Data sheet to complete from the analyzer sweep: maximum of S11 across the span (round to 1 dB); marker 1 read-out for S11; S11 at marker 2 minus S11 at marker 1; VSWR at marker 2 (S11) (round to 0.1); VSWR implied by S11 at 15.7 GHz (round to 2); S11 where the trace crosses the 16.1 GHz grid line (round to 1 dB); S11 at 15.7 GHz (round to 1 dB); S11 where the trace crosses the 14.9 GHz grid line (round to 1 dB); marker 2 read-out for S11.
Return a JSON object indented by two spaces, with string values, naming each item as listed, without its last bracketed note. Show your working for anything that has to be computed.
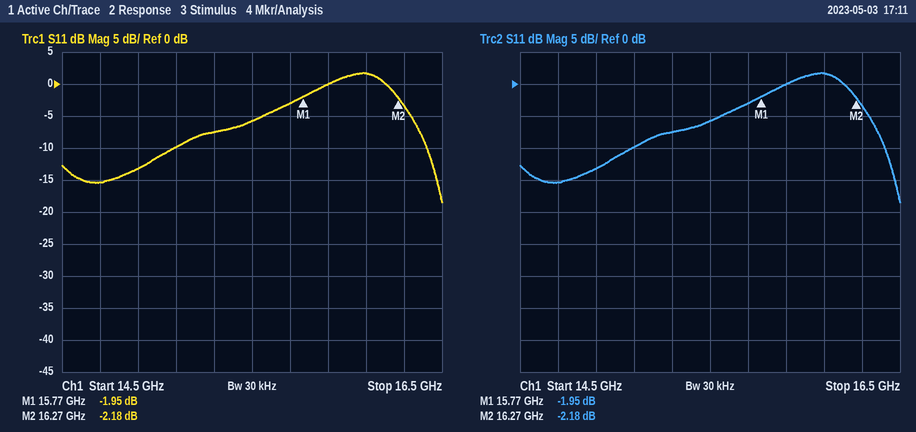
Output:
{
  "maximum of S11 across the span": "2 dB",
  "marker 1 read-out for S11": "-1.95 dB",
  "S11 at marker 2 minus S11 at marker 1": "-2.18 − (-1.95) = -0.23 dB",
  "VSWR at marker 2 (S11)": "(1 + 0.7780)/(1 − 0.7780) ≈ 8.0",
  "VSWR implied by S11 at 15.7 GHz": "|Γ| = 10^(-3/20) = 0.7079; VSWR = (1 + 0.7079)/(1 − 0.7079) ≈ 6",
  "S11 where the trace crosses the 16.1 GHz grid line": "2 dB",
  "S11 at 15.7 GHz": "-3 dB",
  "S11 where the trace crosses the 14.9 GHz grid line": "-13 dB",
  "marker 2 read-out for S11": "-2.18 dB"
}
